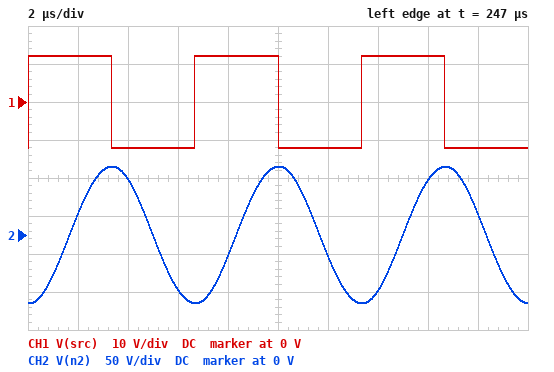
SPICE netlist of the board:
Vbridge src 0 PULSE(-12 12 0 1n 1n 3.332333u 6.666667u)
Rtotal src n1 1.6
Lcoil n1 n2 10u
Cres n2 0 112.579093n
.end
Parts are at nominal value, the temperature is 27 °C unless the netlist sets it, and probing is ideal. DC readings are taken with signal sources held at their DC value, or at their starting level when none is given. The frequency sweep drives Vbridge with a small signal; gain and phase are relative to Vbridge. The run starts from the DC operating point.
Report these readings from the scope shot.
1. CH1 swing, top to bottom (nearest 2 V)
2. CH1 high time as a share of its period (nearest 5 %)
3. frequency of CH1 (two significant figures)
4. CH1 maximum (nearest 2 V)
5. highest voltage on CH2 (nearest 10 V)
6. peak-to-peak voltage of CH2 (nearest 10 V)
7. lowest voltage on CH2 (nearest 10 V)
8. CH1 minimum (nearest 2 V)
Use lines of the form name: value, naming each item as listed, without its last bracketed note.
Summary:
CH1 swing, top to bottom: 24 V
CH1 high time as a share of its period: 50 %
frequency of CH1: 150 kHz
CH1 maximum: 12 V
highest voltage on CH2: 90 V
peak-to-peak voltage of CH2: 180 V
lowest voltage on CH2: -90 V
CH1 minimum: -12 V
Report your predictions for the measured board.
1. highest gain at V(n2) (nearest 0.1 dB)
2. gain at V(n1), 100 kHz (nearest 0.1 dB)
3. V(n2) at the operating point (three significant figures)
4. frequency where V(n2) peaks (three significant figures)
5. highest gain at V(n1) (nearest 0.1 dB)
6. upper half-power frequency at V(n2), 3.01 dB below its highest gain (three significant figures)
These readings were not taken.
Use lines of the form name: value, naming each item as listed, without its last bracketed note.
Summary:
highest gain at V(n2): 15.4 dB
gain at V(n1), 100 kHz: -0.2 dB
V(n2) at the operating point: -12.0 V
frequency where V(n2) peaks: 149 kHz
highest gain at V(n1): 0 dB
upper half-power frequency at V(n2), 3.01 dB below its highest gain: 161 kHz
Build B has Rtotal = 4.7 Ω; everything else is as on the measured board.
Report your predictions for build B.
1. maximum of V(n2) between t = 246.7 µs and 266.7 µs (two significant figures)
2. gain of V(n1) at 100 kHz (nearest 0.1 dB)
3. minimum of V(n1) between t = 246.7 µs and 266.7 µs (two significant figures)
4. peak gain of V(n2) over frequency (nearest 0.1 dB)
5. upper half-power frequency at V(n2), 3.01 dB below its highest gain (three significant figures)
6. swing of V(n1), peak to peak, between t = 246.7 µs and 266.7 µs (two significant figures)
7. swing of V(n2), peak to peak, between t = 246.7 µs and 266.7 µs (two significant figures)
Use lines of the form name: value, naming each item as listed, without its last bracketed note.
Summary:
maximum of V(n2) between t = 246.7 µs and 266.7 µs: 31 V
gain of V(n1) at 100 kHz: -1.3 dB
minimum of V(n1) between t = 246.7 µs and 266.7 µs: -14 V
peak gain of V(n2) over frequency: 6.3 dB
upper half-power frequency at V(n2), 3.01 dB below its highest gain: 175 kHz
swing of V(n1), peak to peak, between t = 246.7 µs and 266.7 µs: 28 V
swing of V(n2), peak to peak, between t = 246.7 µs and 266.7 µs: 62 V
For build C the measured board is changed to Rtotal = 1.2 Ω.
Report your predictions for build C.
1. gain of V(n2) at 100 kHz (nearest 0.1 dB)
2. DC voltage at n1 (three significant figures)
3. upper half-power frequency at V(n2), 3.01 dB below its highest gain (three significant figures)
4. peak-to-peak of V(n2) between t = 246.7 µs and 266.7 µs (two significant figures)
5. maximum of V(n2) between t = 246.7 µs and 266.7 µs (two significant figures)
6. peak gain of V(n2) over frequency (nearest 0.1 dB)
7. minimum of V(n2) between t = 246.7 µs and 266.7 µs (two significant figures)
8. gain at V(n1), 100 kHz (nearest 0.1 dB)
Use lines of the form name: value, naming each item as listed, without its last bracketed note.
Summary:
gain of V(n2) at 100 kHz: 5.0 dB
DC voltage at n1: -12.0 V
upper half-power frequency at V(n2), 3.01 dB below its highest gain: 159 kHz
peak-to-peak of V(n2) between t = 246.7 µs and 266.7 µs: 240 V
maximum of V(n2) between t = 246.7 µs and 266.7 µs: 120 V
peak gain of V(n2) over frequency: 17.9 dB
minimum of V(n2) between t = 246.7 µs and 266.7 µs: -120 V
gain at V(n1), 100 kHz: -0.1 dB
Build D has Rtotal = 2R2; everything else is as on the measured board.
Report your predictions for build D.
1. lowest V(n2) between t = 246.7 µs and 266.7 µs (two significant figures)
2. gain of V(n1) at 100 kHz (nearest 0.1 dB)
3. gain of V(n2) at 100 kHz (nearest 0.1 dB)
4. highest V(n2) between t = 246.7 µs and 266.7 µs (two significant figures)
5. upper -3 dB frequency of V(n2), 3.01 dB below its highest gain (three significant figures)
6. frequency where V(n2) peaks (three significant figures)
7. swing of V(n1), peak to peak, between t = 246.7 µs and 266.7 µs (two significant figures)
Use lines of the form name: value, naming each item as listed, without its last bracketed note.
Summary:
lowest V(n2) between t = 246.7 µs and 266.7 µs: -66 V
gain of V(n1) at 100 kHz: -0.3 dB
gain of V(n2) at 100 kHz: 4.8 dB
highest V(n2) between t = 246.7 µs and 266.7 µs: 66 V
upper -3 dB frequency of V(n2), 3.01 dB below its highest gain: 165 kHz
frequency where V(n2) peaks: 148 kHz
swing of V(n1), peak to peak, between t = 246.7 µs and 266.7 µs: 26 V
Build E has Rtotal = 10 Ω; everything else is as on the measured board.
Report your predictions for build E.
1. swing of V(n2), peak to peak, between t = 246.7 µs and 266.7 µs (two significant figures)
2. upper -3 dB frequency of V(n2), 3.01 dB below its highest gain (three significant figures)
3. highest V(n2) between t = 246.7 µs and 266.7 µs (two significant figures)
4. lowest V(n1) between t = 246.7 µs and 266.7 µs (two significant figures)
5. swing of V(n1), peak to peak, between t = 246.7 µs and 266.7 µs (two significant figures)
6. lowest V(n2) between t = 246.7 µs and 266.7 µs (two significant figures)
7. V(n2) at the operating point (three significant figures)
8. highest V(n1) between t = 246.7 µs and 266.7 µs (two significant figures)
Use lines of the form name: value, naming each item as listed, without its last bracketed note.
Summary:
swing of V(n2), peak to peak, between t = 246.7 µs and 266.7 µs: 30 V
upper -3 dB frequency of V(n2), 3.01 dB below its highest gain: 173 kHz
highest V(n2) between t = 246.7 µs and 266.7 µs: 15 V
lowest V(n1) between t = 246.7 µs and 266.7 µs: -16 V
swing of V(n1), peak to peak, between t = 246.7 µs and 266.7 µs: 31 V
lowest V(n2) between t = 246.7 µs and 266.7 µs: -15 V
V(n2) at the operating point: -12.0 V
highest V(n1) between t = 246.7 µs and 266.7 µs: 16 V
